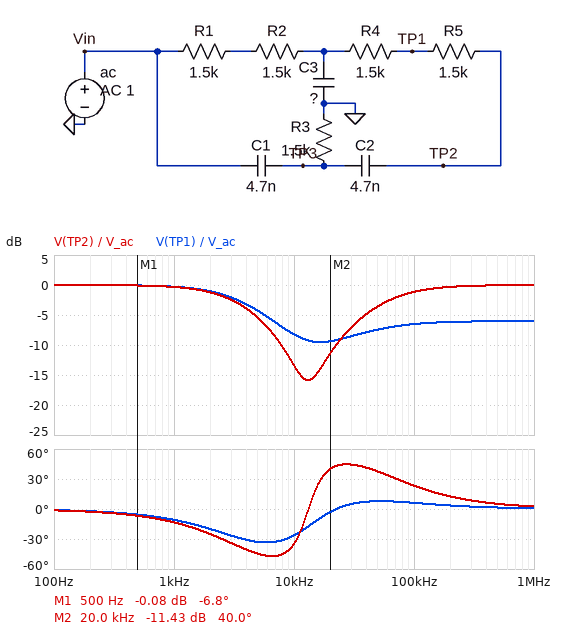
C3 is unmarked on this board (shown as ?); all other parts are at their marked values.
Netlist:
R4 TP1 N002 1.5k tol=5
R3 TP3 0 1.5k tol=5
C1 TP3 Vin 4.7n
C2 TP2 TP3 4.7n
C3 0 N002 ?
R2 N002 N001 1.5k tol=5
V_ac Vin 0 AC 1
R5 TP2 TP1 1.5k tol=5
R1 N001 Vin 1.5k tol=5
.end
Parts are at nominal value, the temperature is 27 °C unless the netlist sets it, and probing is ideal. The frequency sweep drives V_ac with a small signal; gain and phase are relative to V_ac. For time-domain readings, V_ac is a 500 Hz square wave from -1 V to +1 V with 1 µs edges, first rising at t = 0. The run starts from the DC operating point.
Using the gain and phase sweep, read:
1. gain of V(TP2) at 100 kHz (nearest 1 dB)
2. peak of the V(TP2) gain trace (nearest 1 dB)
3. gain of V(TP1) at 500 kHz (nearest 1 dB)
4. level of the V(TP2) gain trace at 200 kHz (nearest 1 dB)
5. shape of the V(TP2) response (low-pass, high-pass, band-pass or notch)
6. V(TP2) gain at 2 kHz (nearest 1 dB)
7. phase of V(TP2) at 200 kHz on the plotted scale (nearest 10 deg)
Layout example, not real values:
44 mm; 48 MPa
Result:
-1 dB; 0 dB; -6 dB; 0 dB; notch; -1 dB; 10 deg
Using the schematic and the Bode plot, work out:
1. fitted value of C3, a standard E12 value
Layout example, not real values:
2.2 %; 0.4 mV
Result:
3.3 nF
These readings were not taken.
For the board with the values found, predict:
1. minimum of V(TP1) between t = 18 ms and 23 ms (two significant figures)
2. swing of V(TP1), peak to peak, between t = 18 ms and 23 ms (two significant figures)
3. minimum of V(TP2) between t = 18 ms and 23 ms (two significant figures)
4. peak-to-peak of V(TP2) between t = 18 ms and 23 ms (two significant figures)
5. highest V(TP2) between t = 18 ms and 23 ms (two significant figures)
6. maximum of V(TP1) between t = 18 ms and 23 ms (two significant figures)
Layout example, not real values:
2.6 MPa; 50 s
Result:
-1.0 V; 2.0 V; -1.0 V; 2.0 V; 1.0 V; 1.0 V
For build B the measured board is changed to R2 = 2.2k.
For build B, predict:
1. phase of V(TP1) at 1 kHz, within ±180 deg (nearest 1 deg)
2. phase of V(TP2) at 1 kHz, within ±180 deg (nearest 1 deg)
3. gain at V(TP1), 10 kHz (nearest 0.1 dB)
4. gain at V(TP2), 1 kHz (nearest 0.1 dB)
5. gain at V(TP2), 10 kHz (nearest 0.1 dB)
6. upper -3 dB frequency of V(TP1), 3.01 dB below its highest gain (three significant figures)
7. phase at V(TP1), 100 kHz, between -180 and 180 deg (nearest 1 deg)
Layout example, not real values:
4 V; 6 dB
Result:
-13 deg; -15 deg; -9.5 dB; -0.4 dB; -15.5 dB; 3.35 kHz; 8 deg
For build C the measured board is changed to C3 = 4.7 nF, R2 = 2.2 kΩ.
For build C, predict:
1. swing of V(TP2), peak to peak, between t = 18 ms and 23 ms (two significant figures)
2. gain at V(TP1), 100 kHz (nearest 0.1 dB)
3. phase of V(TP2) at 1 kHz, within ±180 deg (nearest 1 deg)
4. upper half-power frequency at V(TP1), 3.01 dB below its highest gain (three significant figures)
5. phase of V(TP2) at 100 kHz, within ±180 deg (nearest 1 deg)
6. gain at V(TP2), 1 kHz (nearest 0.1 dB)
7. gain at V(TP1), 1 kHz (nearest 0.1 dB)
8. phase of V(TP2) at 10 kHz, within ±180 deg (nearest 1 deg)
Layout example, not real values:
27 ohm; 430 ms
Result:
2.0 V; -6.8 dB; -17 deg; 3.10 kHz; 24 deg; -0.5 dB; -0.4 dB; -42 deg
